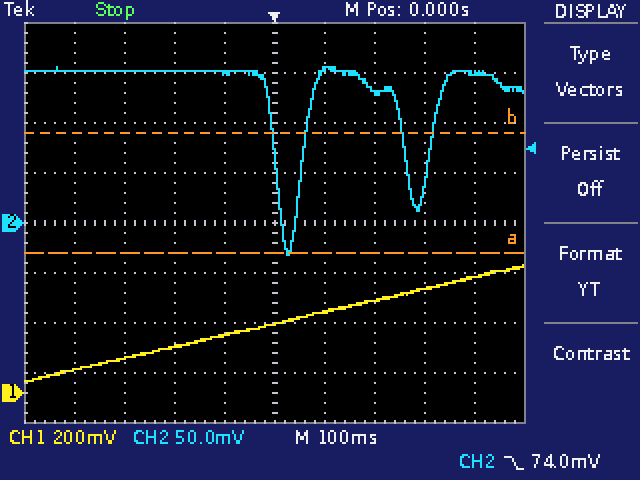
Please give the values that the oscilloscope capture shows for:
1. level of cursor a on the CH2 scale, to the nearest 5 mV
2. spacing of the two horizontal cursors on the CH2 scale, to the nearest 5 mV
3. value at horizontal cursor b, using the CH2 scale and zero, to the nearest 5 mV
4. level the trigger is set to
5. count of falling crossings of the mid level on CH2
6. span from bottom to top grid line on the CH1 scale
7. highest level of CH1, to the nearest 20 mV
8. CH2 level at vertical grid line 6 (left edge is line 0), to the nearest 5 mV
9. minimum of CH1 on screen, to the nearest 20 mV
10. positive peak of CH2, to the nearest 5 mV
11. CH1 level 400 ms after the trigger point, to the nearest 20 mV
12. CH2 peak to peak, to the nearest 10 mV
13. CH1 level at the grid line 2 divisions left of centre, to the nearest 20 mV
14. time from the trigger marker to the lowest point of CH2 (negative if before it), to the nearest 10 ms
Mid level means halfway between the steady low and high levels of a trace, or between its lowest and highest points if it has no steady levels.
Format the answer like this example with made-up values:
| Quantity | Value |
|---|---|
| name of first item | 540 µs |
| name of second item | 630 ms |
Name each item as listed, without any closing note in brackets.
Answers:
| Quantity | Value |
|---|---|
| level of cursor a on the CH2 scale, to the nearest 5 mV | -30 mV |
| spacing of the two horizontal cursors on the CH2 scale, to the nearest 5 mV | 120 mV |
| value at horizontal cursor b, using the CH2 scale and zero, to the nearest 5 mV | 90 mV |
| level the trigger is set to | 74.0 mV |
| count of falling crossings of the mid level on CH2 | 2 |
| span from bottom to top grid line on the CH1 scale | 1.6 V |
| highest level of CH1, to the nearest 20 mV | 520 mV |
| CH2 level at vertical grid line 6 (left edge is line 0), to the nearest 5 mV | 150 mV |
| minimum of CH1 on screen, to the nearest 20 mV | 40 mV |
| positive peak of CH2, to the nearest 5 mV | 155 mV |
| CH1 level 400 ms after the trigger point, to the nearest 20 mV | 460 mV |
| CH2 peak to peak, to the nearest 10 mV | 190 mV |
| CH1 level at the grid line 2 divisions left of centre, to the nearest 20 mV | 180 mV |
| time from the trigger marker to the lowest point of CH2 (negative if before it), to the nearest 10 ms | +30 ms |
